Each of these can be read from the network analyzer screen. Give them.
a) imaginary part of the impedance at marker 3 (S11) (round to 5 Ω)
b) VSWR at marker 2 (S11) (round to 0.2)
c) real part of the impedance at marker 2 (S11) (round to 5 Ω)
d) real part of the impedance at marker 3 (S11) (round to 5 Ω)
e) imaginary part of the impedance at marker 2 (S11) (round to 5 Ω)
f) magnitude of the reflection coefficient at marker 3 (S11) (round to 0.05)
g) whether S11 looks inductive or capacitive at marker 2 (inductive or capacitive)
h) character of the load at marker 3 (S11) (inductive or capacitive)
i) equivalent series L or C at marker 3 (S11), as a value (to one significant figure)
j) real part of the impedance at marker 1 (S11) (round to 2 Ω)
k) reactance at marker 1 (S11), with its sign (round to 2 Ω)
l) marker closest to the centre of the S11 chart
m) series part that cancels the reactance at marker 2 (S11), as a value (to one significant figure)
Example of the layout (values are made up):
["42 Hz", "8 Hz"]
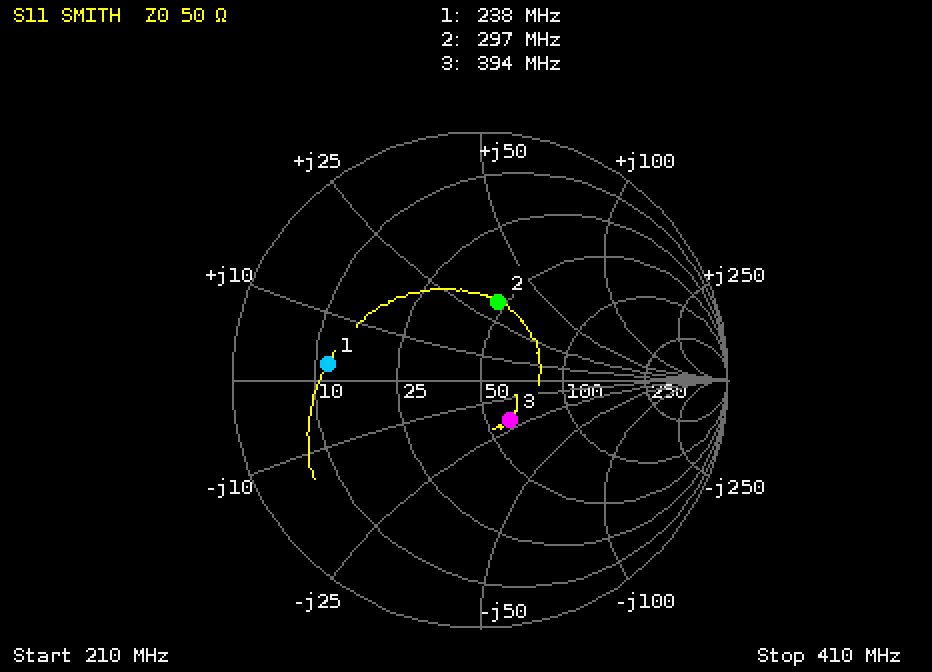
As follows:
["-20 Ω", "2.0", "45 Ω", "60 Ω", "+35 Ω", "0.20", "inductive", "capacitive", "20 pF", "12 Ω", "+2 Ω", "marker 3", "20 pF"]
